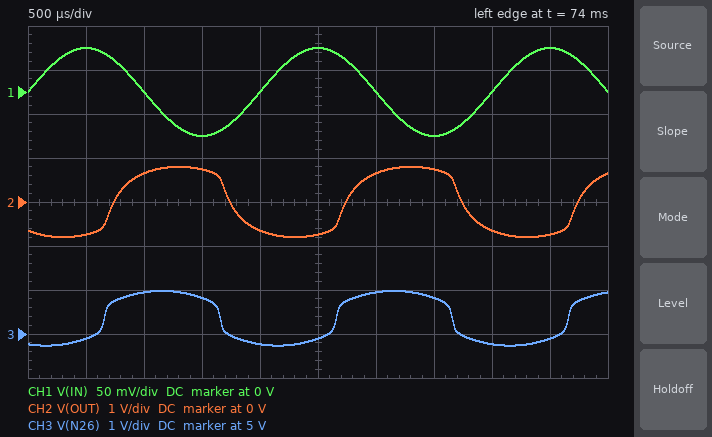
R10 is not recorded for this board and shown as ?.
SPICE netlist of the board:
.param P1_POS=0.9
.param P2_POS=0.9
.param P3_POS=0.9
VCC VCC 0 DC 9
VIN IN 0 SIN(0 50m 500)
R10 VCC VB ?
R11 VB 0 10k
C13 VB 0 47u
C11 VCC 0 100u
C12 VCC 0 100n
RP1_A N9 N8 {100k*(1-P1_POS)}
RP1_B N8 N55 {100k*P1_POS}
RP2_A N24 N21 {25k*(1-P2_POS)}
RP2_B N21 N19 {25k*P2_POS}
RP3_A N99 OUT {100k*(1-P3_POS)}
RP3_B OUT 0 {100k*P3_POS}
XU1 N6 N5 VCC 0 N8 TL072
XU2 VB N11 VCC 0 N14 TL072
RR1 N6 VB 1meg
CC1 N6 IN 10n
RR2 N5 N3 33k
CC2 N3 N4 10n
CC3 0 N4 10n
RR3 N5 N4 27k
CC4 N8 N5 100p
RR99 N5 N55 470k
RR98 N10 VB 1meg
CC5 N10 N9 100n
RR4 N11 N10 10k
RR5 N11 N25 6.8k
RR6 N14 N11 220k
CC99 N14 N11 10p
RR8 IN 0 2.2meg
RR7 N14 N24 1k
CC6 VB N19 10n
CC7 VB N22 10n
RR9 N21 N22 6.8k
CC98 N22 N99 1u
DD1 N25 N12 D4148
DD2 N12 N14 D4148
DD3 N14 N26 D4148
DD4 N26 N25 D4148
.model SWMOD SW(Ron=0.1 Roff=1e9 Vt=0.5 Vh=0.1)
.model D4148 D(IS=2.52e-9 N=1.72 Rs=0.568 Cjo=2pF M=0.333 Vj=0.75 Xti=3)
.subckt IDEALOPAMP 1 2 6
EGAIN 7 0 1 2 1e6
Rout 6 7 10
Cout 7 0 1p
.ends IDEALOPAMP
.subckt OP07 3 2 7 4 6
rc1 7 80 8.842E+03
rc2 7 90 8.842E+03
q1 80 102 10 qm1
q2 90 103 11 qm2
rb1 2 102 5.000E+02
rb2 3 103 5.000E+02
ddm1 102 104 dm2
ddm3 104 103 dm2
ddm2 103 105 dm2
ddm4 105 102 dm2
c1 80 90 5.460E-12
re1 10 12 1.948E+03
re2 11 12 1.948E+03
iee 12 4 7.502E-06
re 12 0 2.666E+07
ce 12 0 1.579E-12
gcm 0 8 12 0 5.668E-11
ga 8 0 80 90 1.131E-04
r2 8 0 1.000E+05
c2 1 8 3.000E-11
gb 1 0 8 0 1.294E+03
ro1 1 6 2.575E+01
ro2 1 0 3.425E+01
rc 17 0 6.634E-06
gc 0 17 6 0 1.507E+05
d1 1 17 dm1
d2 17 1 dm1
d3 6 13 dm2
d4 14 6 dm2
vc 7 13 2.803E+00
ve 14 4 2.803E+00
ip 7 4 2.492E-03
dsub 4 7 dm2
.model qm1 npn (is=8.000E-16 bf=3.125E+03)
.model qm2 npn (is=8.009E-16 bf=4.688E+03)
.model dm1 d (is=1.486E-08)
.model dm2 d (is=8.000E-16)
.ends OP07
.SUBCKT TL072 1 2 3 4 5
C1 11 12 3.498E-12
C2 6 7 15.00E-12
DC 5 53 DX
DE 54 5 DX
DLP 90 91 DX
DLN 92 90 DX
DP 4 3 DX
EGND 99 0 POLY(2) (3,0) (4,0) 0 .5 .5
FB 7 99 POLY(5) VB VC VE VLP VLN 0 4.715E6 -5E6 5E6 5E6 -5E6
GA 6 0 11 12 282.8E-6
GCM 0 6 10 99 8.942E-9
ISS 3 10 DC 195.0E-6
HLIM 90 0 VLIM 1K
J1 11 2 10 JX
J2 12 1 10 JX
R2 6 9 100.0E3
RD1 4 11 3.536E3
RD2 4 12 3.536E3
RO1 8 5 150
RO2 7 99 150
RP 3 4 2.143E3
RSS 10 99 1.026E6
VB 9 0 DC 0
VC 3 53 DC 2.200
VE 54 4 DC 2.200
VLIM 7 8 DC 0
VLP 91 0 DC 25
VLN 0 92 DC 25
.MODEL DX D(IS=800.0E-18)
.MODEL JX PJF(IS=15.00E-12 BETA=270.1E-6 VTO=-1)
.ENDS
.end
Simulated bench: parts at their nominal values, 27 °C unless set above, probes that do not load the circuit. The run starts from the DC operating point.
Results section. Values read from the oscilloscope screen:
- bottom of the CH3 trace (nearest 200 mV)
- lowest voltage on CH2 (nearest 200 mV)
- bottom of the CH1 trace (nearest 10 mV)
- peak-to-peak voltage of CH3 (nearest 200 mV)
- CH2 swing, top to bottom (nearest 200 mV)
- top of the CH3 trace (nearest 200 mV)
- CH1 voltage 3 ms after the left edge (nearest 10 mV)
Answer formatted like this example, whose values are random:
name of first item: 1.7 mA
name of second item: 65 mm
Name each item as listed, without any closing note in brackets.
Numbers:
bottom of the CH3 trace: 4.8 V
lowest voltage on CH2: -800 mV
bottom of the CH1 trace: -50 mV
peak-to-peak voltage of CH3: 1.2 V
CH2 swing, top to bottom: 1.6 V
top of the CH3 trace: 6.0 V
CH1 voltage 3 ms after the left edge: 0 V
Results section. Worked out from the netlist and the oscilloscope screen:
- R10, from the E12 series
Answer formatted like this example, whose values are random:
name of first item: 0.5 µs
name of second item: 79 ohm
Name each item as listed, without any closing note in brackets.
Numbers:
R10, from the E12 series: 6.8 kΩ
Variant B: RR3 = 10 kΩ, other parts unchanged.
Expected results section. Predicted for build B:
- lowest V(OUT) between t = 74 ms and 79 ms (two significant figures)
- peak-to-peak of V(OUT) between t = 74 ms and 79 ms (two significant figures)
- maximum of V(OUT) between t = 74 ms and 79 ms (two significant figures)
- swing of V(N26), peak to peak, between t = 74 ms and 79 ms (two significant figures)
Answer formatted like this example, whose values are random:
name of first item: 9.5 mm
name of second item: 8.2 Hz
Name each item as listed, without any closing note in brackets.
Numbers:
lowest V(OUT) between t = 74 ms and 79 ms: -840 mV
peak-to-peak of V(OUT) between t = 74 ms and 79 ms: 1.7 V
maximum of V(OUT) between t = 74 ms and 79 ms: 840 mV
swing of V(N26), peak to peak, between t = 74 ms and 79 ms: 1.3 V
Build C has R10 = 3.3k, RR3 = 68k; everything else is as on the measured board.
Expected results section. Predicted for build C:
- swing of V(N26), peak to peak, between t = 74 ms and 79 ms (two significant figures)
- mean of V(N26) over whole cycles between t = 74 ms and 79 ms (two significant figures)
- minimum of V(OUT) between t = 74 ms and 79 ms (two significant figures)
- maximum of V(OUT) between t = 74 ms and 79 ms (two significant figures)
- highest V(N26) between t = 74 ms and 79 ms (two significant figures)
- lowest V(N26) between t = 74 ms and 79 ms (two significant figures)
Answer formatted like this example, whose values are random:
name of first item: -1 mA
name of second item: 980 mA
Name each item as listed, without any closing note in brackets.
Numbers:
swing of V(N26), peak to peak, between t = 74 ms and 79 ms: 850 mV
mean of V(N26) over whole cycles between t = 74 ms and 79 ms: 6.7 V
minimum of V(OUT) between t = 74 ms and 79 ms: -700 mV
maximum of V(OUT) between t = 74 ms and 79 ms: 550 mV
highest V(N26) between t = 74 ms and 79 ms: 7.1 V
lowest V(N26) between t = 74 ms and 79 ms: 6.2 V
